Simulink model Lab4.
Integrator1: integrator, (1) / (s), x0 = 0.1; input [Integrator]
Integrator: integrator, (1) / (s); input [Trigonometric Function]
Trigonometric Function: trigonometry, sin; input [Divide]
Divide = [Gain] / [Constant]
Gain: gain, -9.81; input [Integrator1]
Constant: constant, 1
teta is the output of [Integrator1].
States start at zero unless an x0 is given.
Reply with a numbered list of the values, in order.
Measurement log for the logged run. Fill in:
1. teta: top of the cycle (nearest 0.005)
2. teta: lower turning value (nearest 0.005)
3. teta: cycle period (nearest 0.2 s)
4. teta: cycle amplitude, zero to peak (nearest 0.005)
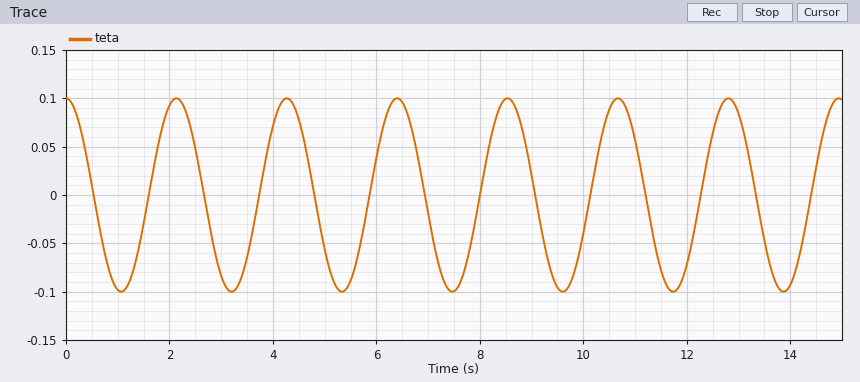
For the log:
1. 0.100
2. -0.100
3. 2.2 s
4. 0.100
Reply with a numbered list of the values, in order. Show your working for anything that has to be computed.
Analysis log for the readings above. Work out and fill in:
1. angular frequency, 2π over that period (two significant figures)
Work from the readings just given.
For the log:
1. 2π / 2.2 = 2.9 rad/s
